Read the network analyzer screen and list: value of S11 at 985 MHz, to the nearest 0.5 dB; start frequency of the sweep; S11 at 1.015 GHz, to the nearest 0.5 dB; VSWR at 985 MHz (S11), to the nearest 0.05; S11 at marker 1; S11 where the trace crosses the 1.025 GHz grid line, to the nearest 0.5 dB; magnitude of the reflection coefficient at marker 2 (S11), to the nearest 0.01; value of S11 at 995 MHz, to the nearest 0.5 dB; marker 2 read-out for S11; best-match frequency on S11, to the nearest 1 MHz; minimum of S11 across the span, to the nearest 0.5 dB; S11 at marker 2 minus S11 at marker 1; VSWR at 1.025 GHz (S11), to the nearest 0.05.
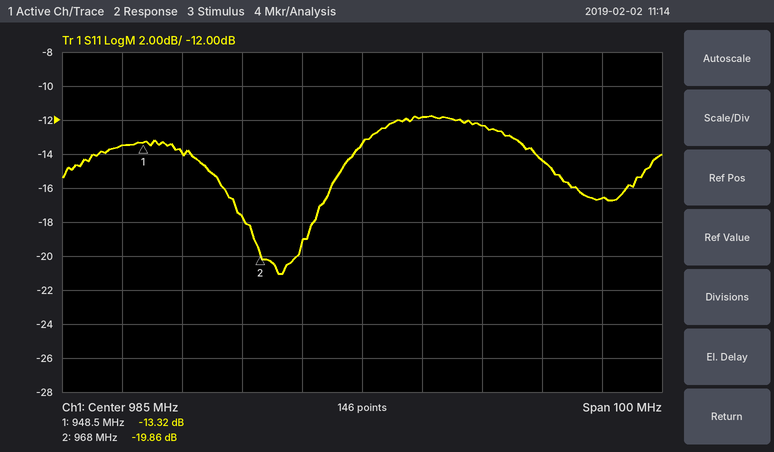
-13.5 dB
935 MHz
-14.5 dB
1.55
-13.32 dB
-16.5 dB
0.10
-12.0 dB
-19.86 dB
971 MHz
-21.0 dB
-6.54 dB
1.35
